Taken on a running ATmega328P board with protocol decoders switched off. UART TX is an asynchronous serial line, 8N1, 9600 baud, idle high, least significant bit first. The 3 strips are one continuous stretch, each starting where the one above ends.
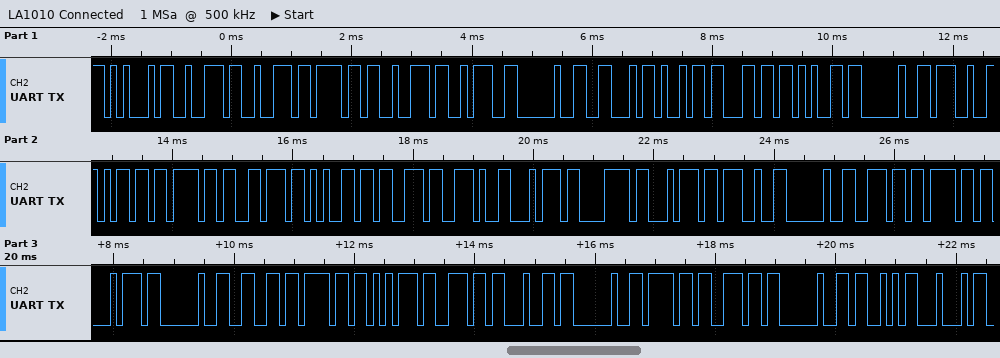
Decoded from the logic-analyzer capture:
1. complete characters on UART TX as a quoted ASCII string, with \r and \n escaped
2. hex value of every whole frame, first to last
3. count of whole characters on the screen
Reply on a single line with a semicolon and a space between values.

"Error: File 'moves.txt' not found on SD"; 45 72 72 6F 72 3A 20 46 69 6C 65 20 27 6D 6F 76 65 73 2E 74 78 74 27 20 6E 6F 74 20 66 6F 75 6E 64 20 6F 6E 20 53 44; 39
